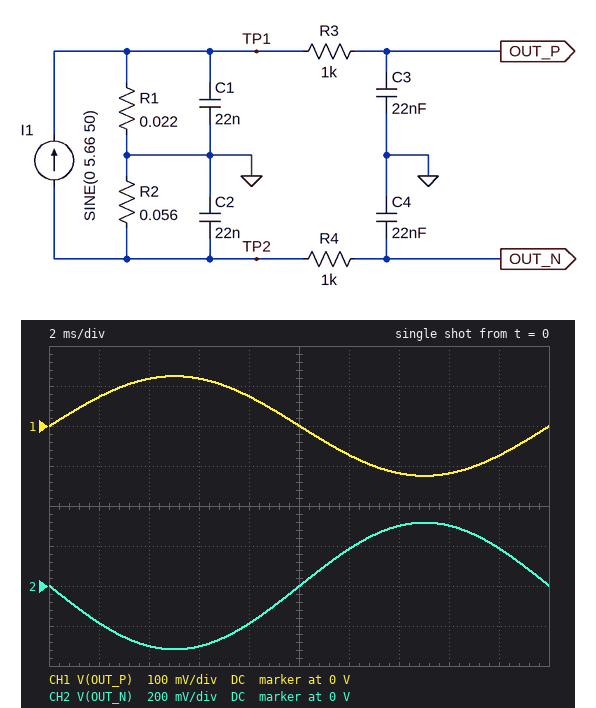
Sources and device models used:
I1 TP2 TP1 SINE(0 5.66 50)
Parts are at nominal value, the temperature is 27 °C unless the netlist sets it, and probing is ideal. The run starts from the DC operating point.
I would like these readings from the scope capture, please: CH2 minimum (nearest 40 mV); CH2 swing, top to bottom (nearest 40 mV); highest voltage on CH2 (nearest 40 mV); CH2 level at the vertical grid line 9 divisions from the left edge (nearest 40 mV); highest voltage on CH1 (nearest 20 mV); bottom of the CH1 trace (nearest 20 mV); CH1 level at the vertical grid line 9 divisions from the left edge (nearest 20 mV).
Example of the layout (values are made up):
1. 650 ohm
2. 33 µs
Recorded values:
1. -320 mV
2. 640 mV
3. 320 mV
4. 200 mV
5. 120 mV
6. -120 mV
7. -80 mV
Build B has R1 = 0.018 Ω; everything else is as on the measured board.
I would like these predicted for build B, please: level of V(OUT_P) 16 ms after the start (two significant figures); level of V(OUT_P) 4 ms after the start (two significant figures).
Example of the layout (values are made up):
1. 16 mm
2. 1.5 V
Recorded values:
1. -97 mV
2. 97 mV
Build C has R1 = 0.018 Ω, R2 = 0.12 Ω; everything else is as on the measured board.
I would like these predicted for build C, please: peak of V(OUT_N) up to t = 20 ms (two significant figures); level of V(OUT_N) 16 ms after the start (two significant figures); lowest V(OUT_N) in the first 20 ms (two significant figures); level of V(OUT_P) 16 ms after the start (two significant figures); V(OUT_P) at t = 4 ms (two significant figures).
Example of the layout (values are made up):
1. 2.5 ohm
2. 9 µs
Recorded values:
1. 680 mV
2. 650 mV
3. -680 mV
4. -97 mV
5. 97 mV
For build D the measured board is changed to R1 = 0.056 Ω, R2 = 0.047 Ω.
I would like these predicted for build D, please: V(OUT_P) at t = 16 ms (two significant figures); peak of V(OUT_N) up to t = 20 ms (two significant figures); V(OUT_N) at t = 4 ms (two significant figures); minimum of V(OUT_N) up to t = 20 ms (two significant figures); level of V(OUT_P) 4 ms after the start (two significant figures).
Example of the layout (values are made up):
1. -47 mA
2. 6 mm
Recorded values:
1. -300 mV
2. 270 mV
3. -250 mV
4. -270 mV
5. 300 mV
